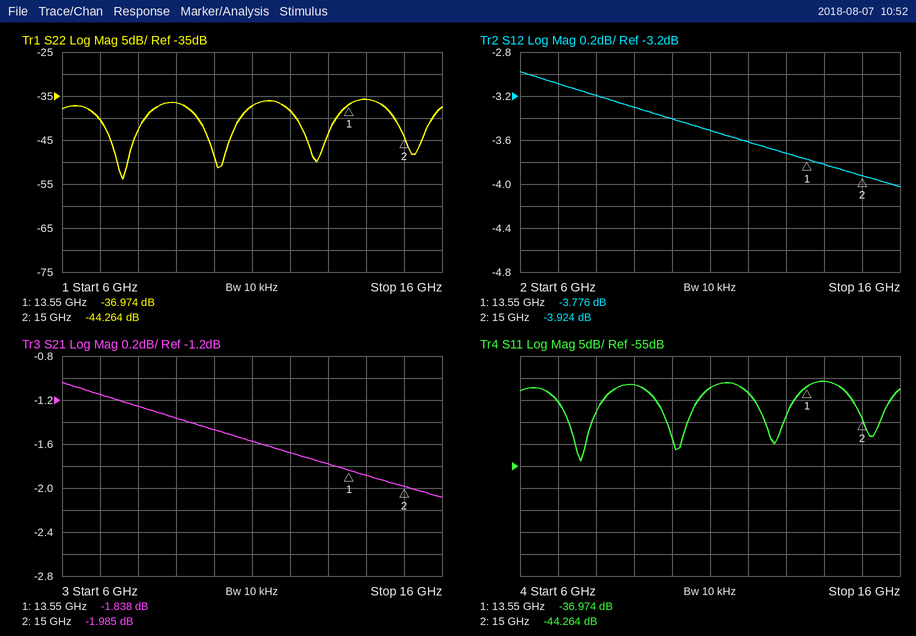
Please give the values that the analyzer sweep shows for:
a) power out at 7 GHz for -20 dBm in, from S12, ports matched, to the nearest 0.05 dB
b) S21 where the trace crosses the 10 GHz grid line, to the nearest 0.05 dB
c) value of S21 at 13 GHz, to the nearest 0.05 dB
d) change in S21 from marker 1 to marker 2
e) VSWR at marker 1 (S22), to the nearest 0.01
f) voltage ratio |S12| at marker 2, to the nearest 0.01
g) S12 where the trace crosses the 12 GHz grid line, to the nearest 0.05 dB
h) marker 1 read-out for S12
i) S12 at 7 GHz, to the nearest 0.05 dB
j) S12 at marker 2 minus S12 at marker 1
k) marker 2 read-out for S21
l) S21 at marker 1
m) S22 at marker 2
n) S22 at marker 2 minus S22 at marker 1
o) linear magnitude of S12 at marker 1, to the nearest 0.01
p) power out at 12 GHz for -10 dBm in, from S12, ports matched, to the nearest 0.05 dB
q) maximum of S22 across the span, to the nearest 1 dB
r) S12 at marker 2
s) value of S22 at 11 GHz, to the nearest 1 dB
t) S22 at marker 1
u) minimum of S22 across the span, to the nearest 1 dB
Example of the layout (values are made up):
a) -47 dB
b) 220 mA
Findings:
a) -23.10 dBm
b) -1.45 dB
c) -1.80 dB
d) -0.147 dB
e) 1.03
f) 0.64
g) -3.60 dB
h) -3.776 dB
i) -3.10 dB
j) -0.148 dB
k) -1.985 dB
l) -1.838 dB
m) -44.264 dB
n) -7.290 dB
o) 0.65
p) -13.60 dBm
q) -36 dB
r) -3.924 dB
s) -37 dB
t) -36.974 dB
u) -54 dB
